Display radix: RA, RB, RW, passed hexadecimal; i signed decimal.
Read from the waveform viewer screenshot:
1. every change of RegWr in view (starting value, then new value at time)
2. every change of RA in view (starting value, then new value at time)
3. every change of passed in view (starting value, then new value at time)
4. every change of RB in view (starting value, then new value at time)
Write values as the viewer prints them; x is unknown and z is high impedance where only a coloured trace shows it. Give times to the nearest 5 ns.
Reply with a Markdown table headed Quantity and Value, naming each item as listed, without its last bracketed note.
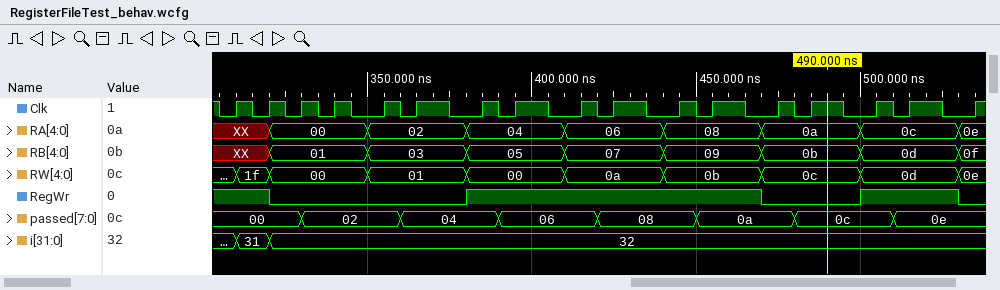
| Quantity | Value |
|---|---|
| every change of RegWr in view | 1, 0 at 320 ns, 1 at 380 ns, 0 at 470 ns, 1 at 500 ns, 0 at 530 ns |
| every change of RA in view | XX, 00 at 320 ns, 02 at 350 ns, 04 at 380 ns, 06 at 410 ns, 08 at 440 ns, 0a at 470 ns, 0c at 500 ns, 0e at 530 ns |
| every change of passed in view | 00, 02 at 330 ns, 04 at 360 ns, 06 at 390 ns, 08 at 420 ns, 0a at 450 ns, 0c at 480 ns, 0e at 510 ns |
| every change of RB in view | XX, 01 at 320 ns, 03 at 350 ns, 05 at 380 ns, 07 at 410 ns, 09 at 440 ns, 0b at 470 ns, 0d at 500 ns, 0f at 530 ns |
